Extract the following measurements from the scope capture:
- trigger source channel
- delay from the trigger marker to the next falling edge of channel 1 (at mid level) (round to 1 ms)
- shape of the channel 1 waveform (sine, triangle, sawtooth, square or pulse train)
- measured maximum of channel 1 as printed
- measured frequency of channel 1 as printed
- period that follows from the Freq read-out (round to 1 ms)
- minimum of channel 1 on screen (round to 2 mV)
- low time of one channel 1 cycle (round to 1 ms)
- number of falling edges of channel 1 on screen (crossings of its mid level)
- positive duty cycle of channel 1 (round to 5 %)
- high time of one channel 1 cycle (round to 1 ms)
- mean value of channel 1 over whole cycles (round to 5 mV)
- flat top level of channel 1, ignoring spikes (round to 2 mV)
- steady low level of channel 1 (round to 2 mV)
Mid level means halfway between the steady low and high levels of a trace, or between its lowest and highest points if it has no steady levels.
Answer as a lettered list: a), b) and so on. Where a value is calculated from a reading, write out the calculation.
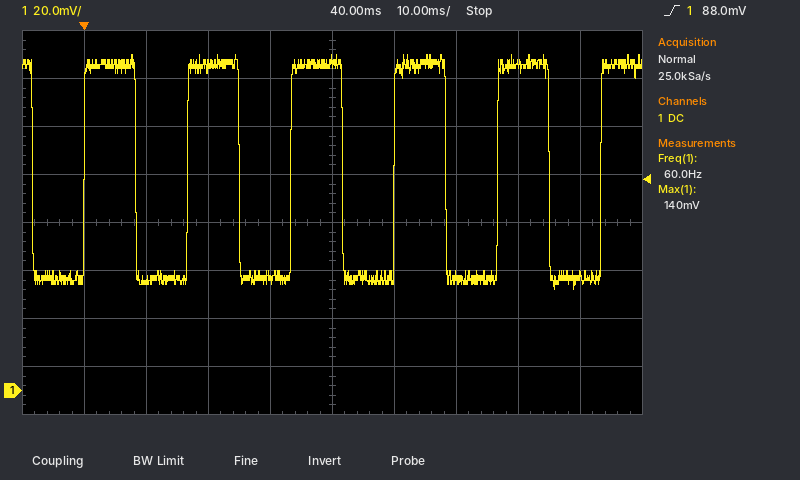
a) channel 1
b) 8 ms
c) square
d) 140 mV
e) 60.0 Hz
f) 1 / 60.0 Hz ≈ 17 ms
g) 42 mV
h) 8 ms
i) 6
j) 50 %
k) 8 ms
l) 46 mV + 0.5 × (136 mV − (46 mV)) ≈ 91.0 mV, so 90 mV to the nearest 5 mV
m) 136 mV
n) 46 mV
